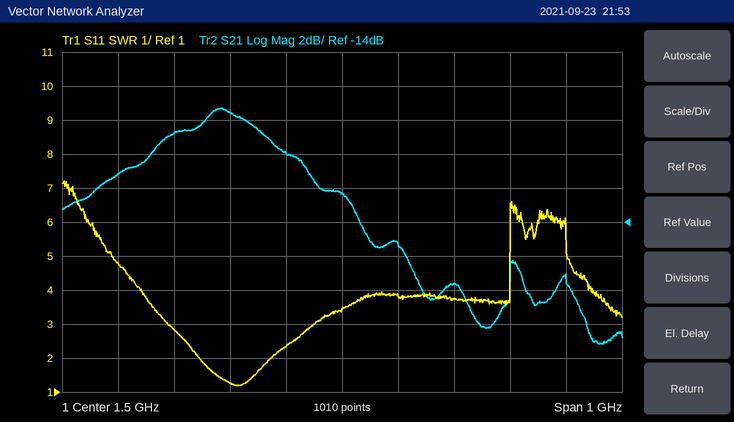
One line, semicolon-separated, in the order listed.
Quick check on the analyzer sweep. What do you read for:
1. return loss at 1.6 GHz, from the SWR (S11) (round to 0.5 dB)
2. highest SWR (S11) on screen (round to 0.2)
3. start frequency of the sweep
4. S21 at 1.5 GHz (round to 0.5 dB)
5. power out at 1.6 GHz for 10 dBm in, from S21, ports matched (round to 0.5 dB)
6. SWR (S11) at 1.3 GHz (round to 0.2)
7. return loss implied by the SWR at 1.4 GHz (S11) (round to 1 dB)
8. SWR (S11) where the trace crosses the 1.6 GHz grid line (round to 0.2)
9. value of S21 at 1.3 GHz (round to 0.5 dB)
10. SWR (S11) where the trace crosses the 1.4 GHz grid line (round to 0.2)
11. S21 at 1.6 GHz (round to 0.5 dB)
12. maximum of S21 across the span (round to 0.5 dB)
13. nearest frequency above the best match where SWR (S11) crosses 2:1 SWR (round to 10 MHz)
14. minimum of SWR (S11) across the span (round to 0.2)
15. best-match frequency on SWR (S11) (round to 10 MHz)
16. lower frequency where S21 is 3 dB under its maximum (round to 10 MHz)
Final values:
4.5 dB; 7.2; 1 GHz; -12.5 dB; -5.5 dBm; 1.2; 8 dB; 3.8; -7.5 dB; 2.4; -15.5 dB; -7.5 dB; 1.37 GHz; 1.2; 1.31 GHz; 1.15 GHz
